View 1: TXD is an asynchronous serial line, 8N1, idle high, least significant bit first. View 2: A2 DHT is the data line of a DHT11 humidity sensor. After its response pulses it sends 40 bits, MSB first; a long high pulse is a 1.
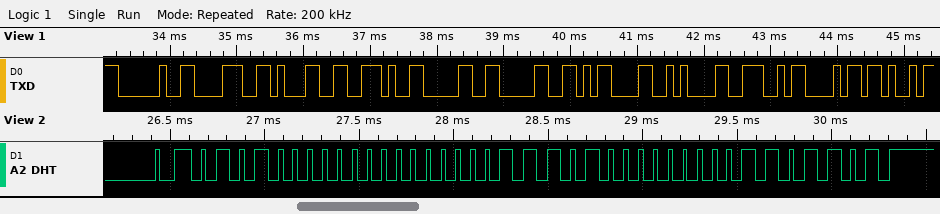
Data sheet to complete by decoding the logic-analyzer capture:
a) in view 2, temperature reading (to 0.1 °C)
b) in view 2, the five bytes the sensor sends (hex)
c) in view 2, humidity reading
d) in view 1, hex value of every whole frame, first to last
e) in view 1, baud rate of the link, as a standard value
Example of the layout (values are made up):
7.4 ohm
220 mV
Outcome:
29.0 °C
50 00 1D 00 6D
80 %
0x20 0x38 0x31 0x2E 0x30 0x30 0x0D 0x0A 0x4E 0x68
9600 baud
